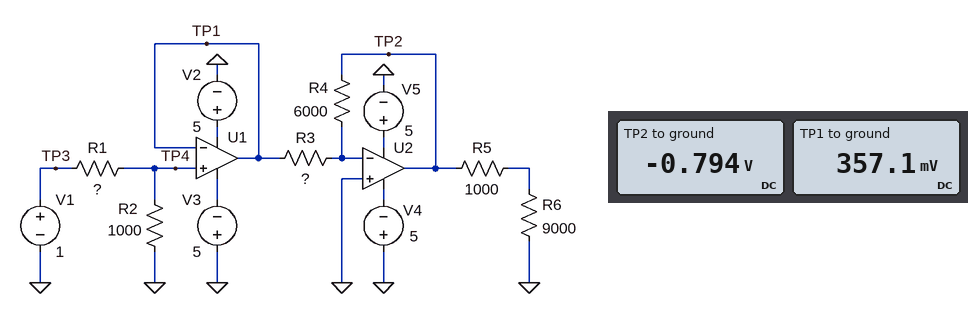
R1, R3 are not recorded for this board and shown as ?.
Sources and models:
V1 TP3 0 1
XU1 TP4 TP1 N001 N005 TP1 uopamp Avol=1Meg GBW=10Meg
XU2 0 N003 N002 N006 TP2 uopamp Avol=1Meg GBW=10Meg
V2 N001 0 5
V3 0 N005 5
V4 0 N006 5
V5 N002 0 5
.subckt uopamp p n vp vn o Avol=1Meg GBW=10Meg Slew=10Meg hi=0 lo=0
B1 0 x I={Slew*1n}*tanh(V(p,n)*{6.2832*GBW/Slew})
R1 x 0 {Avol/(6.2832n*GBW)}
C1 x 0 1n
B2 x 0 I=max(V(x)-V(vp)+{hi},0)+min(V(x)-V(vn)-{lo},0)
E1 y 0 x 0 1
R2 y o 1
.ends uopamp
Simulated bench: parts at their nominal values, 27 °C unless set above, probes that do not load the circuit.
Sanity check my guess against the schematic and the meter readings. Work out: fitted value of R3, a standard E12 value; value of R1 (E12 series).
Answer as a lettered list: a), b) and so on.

a) 2.7 kΩ
b) 1.8 kΩ
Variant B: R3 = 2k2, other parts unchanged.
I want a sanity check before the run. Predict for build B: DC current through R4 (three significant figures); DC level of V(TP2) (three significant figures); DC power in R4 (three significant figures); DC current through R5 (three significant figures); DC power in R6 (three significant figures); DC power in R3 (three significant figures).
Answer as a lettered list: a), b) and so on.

a) 162 µA
b) -974 mV
c) 158 µW
d) 97.4 µA
e) 85.4 µW
f) 58.0 µW
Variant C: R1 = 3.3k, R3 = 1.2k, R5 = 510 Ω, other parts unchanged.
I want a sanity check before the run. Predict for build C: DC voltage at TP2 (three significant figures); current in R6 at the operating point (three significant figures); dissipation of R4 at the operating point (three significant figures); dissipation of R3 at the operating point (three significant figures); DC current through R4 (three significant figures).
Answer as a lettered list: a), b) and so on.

a) -1.16 V
b) 122 µA
c) 225 µW
d) 45.1 µW
e) 194 µA
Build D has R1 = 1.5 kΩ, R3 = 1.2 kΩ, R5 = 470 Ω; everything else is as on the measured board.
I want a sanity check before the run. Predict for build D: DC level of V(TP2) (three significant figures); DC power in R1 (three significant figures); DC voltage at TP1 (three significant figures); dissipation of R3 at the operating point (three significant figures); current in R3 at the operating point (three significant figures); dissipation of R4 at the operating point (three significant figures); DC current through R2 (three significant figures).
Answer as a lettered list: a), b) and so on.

a) -2.00 V
b) 240 µW
c) 400 mV
d) 133 µW
e) 333 µA
f) 667 µW
g) 400 µA
